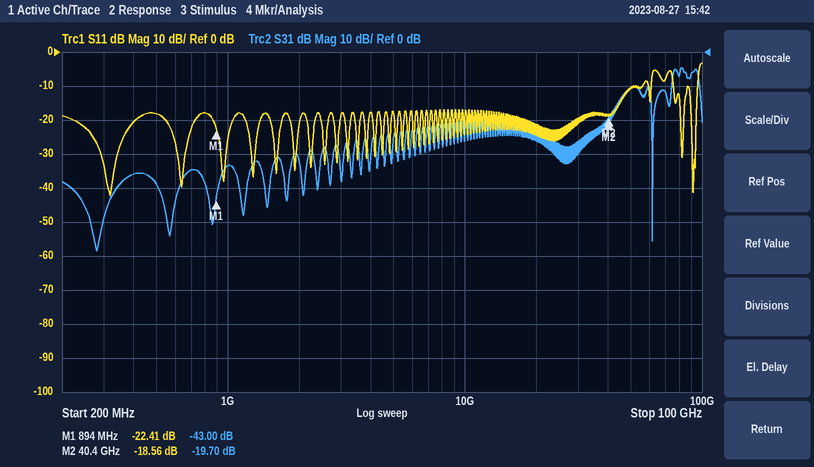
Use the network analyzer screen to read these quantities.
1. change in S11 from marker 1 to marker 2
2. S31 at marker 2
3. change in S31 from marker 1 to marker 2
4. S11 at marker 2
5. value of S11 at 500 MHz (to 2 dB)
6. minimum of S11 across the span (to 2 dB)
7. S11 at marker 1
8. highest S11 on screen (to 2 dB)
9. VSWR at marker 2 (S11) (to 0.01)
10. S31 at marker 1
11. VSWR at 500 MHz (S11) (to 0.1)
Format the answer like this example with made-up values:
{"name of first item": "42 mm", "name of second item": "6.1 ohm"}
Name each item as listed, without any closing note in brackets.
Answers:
{"change in S11 from marker 1 to marker 2": "3.85 dB", "S31 at marker 2": "-19.70 dB", "change in S31 from marker 1 to marker 2": "23.30 dB", "S11 at marker 2": "-18.56 dB", "value of S11 at 500 MHz": "-18 dB", "minimum of S11 across the span": "-42 dB", "S11 at marker 1": "-22.41 dB", "highest S11 on screen": "-4 dB", "VSWR at marker 2 (S11)": "1.27", "S31 at marker 1": "-43.00 dB", "VSWR at 500 MHz (S11)": "1.3"}
